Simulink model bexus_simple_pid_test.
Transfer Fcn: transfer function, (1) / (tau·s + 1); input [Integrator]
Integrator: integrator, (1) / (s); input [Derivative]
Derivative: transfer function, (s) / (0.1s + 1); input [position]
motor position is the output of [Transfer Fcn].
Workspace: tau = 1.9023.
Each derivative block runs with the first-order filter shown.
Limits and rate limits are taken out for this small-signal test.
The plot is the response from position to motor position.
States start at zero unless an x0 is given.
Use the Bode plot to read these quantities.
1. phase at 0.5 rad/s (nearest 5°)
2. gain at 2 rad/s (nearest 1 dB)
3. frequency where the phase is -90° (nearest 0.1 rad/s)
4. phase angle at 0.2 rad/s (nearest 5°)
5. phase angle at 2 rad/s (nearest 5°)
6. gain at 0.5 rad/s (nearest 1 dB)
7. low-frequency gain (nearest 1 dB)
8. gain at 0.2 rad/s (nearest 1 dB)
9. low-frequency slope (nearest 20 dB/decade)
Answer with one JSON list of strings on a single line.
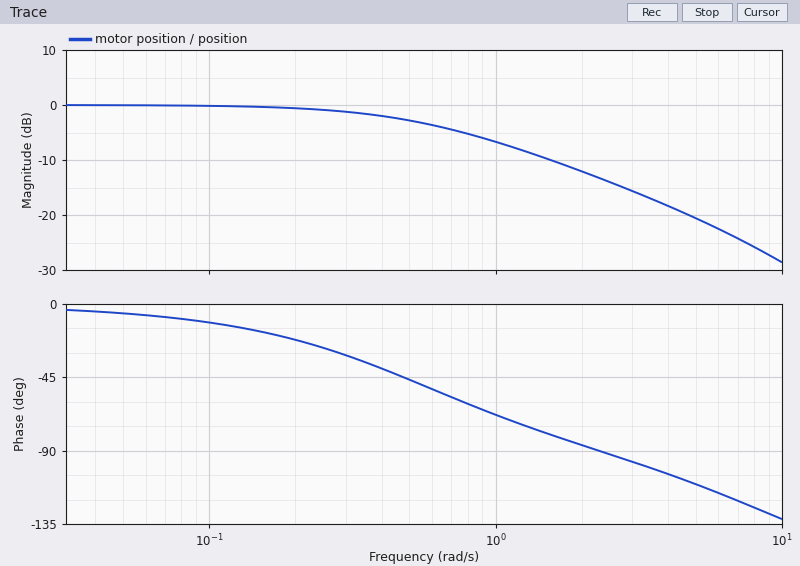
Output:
["-45°", "-12 dB", "2.3 rad/s", "-20°", "-85°", "-3 dB", "0 dB", "-1 dB", "0 dB/decade"]
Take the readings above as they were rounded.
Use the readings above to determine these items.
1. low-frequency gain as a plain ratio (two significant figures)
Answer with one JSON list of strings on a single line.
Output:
["1.0"]
